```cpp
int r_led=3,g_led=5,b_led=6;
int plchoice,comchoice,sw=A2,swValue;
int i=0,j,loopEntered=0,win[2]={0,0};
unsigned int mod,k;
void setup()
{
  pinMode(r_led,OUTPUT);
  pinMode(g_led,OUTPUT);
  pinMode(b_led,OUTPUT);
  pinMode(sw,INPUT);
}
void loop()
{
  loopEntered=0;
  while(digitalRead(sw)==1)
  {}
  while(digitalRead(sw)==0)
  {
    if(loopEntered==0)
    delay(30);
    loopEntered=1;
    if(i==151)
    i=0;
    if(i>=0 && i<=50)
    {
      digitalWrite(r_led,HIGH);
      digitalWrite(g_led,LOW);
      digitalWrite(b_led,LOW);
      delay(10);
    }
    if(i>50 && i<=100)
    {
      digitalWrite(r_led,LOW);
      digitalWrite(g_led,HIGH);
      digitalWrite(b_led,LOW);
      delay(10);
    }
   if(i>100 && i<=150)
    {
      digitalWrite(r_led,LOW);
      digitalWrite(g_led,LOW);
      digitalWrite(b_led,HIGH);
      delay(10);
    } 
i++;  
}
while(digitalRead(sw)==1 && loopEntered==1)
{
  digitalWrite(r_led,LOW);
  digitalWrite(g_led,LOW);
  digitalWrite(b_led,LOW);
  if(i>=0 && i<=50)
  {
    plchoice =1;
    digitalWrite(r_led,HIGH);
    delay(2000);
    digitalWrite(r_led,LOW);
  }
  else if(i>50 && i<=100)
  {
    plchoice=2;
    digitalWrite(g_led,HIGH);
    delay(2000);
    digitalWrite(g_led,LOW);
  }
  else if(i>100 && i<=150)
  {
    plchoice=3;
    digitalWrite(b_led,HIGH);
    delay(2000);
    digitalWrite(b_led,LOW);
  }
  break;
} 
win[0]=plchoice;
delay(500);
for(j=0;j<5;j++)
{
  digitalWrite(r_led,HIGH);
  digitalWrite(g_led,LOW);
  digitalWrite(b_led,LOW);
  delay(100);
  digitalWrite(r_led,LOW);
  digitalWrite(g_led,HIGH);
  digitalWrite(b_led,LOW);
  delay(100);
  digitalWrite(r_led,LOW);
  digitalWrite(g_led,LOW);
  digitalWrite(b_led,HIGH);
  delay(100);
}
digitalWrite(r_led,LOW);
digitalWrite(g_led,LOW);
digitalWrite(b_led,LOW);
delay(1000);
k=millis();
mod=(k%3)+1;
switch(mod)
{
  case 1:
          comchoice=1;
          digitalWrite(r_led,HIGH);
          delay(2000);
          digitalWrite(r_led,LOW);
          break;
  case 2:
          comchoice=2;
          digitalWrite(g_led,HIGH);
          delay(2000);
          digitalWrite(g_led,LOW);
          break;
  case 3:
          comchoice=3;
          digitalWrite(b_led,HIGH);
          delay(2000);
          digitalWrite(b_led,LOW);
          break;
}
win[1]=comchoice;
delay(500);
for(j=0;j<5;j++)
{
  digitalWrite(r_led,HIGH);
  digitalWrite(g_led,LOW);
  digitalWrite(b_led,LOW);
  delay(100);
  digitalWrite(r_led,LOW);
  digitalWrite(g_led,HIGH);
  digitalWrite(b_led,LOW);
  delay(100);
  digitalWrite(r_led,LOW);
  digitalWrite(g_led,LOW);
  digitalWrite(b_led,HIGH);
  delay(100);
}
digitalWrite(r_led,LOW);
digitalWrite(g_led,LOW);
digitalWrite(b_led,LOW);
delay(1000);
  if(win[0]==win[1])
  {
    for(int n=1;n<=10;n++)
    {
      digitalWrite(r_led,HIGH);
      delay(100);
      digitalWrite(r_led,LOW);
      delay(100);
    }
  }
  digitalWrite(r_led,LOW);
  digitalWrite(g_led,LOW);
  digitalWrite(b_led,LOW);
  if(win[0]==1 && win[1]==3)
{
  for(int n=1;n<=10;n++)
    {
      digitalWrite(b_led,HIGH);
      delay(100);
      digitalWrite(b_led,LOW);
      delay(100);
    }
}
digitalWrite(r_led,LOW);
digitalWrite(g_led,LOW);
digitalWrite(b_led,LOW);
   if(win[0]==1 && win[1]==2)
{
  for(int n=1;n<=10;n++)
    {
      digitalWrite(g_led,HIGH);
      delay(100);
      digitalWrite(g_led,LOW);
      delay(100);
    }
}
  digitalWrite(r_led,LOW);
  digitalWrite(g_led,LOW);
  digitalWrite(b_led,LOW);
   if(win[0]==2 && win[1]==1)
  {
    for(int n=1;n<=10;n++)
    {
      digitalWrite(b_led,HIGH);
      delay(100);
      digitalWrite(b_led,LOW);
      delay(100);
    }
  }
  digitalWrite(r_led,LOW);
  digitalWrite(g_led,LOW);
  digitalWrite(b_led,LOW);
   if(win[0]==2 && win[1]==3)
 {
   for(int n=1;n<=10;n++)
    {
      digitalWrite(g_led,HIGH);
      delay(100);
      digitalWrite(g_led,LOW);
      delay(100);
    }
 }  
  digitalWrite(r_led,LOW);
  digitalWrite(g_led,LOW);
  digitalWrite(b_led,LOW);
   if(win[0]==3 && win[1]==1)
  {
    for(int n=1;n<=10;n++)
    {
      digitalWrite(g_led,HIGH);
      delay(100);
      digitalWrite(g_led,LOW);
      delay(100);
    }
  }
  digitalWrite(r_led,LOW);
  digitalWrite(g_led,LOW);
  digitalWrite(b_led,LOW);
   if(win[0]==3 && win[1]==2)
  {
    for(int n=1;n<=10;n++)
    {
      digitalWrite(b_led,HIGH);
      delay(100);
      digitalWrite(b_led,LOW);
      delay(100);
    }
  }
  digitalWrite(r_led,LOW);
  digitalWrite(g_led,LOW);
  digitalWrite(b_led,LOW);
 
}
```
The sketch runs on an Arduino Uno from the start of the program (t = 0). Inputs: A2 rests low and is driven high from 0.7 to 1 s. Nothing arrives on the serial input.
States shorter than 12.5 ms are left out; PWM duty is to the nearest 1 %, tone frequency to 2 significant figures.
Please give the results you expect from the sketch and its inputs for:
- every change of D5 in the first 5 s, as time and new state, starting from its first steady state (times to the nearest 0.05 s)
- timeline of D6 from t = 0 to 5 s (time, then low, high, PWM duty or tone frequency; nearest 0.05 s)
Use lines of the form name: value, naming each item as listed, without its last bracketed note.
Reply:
every change of D5 in the first 5 s, as time and new state, starting from its first steady state: 0 s low; 0.55 s high; 2.7 s low; 3.3 s high; 3.4 s low; 3.6 s high; 3.7 s low; 3.9 s high; 4 s low; 4.2 s high; 4.3 s low; 4.5 s high; 4.6 s low
timeline of D6 from t = 0 to 5 s: 0 s low; 3.4 s high; 3.5 s low; 3.7 s high; 3.8 s low; 4 s high; 4.1 s low; 4.3 s high; 4.4 s low; 4.6 s high; 4.7 s low
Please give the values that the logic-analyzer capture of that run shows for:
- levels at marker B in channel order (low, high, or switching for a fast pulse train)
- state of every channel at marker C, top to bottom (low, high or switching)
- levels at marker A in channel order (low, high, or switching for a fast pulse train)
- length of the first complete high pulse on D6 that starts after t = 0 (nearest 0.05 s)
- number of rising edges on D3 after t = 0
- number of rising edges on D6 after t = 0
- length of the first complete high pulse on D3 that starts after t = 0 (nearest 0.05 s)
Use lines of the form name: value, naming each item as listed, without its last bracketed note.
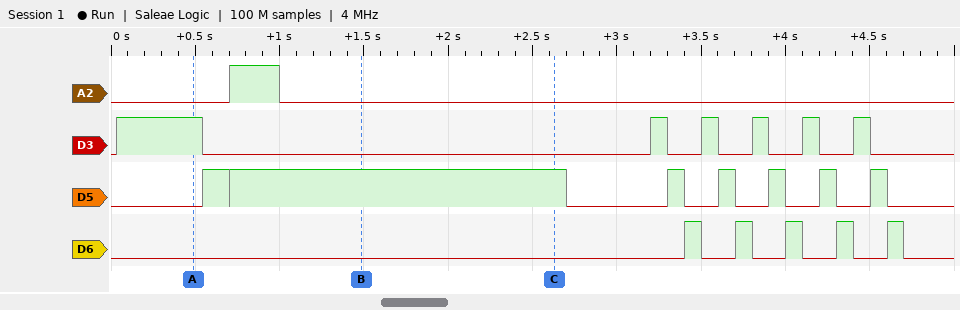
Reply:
levels at marker B in channel order: A2 low, D3 low, D5 high, D6 low
state of every channel at marker C, top to bottom: A2 low, D3 low, D5 high, D6 low
levels at marker A in channel order: A2 low, D3 high, D5 low, D6 low
length of the first complete high pulse on D6 that starts after t = 0: 0.10 s
number of rising edges on D3 after t = 0: 6
number of rising edges on D6 after t = 0: 5
length of the first complete high pulse on D3 that starts after t = 0: 0.50 s
